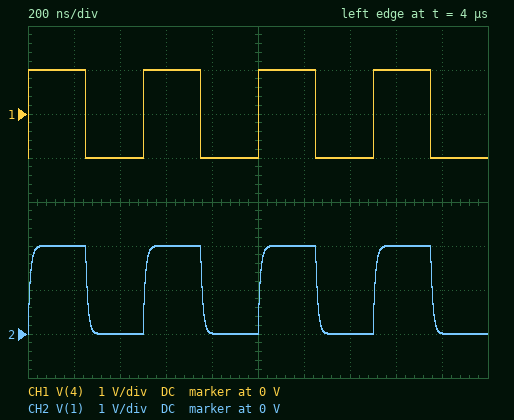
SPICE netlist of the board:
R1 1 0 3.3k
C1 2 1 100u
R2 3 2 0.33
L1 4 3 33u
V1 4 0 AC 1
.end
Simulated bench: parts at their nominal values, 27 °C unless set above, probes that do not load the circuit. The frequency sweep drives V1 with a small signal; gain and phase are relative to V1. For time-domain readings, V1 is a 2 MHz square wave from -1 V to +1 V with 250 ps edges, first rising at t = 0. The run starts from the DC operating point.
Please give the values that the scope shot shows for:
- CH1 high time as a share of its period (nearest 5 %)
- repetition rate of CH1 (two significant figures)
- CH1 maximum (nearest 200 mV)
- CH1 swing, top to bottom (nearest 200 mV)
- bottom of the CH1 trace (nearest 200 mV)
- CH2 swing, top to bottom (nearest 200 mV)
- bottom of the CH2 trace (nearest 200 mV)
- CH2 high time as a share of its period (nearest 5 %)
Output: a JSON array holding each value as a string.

["50 %", "2.0 MHz", "1.0 V", "2.0 V", "-1.0 V", "2.0 V", "0 V", "50 %"]
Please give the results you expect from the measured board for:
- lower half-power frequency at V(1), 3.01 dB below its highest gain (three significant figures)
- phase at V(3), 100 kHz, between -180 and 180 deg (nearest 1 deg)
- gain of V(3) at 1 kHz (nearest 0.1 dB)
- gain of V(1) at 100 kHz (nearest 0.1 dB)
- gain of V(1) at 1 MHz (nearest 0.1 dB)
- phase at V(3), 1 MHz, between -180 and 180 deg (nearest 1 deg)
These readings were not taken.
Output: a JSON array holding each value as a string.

["482 mHz", "0 deg", "0 dB", "0 dB", "0 dB", "-4 deg"]
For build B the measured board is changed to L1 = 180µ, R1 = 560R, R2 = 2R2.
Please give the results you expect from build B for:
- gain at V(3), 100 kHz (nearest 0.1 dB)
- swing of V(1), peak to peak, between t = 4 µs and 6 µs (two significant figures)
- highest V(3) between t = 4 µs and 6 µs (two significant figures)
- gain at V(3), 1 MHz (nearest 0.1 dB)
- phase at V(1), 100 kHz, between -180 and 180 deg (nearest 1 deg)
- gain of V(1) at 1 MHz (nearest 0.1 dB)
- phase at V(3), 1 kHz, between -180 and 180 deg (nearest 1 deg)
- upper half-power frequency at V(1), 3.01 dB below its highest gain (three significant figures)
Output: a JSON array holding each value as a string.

["-0.2 dB", "740 mV", "370 mV", "-7.0 dB", "-11 deg", "-7.1 dB", "0 deg", "497 kHz"]
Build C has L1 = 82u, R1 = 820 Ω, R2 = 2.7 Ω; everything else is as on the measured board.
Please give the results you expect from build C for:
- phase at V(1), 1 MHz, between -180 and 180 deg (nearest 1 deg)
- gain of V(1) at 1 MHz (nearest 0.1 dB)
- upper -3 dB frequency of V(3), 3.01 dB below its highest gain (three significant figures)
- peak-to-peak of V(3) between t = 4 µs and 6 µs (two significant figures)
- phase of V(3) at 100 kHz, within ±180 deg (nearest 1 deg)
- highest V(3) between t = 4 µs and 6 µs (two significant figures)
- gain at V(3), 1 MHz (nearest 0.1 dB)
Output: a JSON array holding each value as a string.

["-32 deg", "-1.5 dB", "1.60 MHz", "1.7 V", "-4 deg", "850 mV", "-1.4 dB"]
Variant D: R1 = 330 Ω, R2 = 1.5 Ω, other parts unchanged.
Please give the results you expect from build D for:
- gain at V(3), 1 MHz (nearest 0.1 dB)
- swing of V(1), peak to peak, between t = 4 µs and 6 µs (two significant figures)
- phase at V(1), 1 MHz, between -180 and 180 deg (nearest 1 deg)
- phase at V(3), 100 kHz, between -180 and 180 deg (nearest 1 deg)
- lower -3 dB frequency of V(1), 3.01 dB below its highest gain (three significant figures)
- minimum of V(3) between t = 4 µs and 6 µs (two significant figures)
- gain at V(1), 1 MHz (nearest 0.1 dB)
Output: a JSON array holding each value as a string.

["-1.4 dB", "1.7 V", "-32 deg", "-4 deg", "4.80 Hz", "-850 mV", "-1.5 dB"]
